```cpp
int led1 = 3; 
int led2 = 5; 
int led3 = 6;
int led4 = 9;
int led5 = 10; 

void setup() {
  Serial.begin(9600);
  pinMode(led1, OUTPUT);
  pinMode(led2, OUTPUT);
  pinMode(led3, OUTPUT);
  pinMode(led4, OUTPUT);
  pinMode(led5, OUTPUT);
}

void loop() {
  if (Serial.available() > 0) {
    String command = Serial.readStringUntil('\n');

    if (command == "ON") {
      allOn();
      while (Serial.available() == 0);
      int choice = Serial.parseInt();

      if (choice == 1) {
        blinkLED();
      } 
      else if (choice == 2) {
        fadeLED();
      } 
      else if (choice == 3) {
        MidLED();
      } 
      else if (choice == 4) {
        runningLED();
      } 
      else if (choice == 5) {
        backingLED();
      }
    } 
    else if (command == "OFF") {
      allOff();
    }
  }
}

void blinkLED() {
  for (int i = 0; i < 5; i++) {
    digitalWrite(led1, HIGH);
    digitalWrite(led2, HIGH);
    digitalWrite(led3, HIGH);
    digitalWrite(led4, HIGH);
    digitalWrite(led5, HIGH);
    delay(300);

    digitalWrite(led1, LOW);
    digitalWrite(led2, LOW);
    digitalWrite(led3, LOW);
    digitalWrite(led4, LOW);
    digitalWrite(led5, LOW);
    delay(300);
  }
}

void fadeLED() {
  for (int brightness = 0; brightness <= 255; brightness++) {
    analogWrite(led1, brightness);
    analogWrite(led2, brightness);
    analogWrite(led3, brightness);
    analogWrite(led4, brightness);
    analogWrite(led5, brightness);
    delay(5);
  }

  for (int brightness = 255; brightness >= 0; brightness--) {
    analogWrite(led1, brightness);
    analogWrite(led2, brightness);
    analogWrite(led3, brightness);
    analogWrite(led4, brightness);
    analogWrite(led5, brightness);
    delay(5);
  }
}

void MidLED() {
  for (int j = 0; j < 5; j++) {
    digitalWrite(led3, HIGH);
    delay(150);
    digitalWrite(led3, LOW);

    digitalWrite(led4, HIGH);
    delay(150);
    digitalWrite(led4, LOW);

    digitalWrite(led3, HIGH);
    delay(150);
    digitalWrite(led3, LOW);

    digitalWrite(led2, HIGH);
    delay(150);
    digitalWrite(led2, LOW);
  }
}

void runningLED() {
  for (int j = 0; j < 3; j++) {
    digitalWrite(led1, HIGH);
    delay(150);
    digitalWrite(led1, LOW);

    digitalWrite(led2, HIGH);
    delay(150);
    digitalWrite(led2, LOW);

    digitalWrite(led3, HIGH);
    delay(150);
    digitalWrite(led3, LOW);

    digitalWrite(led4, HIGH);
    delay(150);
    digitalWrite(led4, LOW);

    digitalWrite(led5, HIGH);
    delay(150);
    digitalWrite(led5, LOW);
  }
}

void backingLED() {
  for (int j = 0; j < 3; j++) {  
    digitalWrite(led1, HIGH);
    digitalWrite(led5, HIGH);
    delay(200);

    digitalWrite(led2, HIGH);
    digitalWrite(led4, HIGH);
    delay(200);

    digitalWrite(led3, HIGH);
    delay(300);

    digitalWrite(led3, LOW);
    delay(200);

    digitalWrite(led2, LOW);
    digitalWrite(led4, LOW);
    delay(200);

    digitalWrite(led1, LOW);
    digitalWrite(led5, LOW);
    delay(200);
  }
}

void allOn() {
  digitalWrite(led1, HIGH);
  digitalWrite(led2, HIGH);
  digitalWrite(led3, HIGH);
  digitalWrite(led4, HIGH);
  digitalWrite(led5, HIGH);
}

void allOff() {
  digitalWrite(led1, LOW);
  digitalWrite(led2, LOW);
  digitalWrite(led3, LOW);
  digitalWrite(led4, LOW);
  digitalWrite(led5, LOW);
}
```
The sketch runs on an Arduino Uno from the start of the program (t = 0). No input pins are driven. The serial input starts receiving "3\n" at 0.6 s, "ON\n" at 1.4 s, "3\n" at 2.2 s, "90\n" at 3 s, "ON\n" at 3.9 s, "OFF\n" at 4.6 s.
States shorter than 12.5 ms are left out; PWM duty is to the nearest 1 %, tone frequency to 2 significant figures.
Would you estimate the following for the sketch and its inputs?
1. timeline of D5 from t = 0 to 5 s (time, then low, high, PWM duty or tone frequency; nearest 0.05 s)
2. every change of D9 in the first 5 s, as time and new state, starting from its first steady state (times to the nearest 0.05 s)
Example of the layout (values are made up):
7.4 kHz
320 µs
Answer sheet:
0 s low; 1.4 s high; 2.8 s low; 3.25 s high; 3.4 s low; 3.85 s high; 4 s low; 4.45 s high; 4.6 s low
0 s low; 1.4 s high; 2.5 s low; 2.95 s high; 3.1 s low; 3.55 s high; 3.7 s low; 4.15 s high; 4.3 s low; 4.75 s high; 4.9 s low
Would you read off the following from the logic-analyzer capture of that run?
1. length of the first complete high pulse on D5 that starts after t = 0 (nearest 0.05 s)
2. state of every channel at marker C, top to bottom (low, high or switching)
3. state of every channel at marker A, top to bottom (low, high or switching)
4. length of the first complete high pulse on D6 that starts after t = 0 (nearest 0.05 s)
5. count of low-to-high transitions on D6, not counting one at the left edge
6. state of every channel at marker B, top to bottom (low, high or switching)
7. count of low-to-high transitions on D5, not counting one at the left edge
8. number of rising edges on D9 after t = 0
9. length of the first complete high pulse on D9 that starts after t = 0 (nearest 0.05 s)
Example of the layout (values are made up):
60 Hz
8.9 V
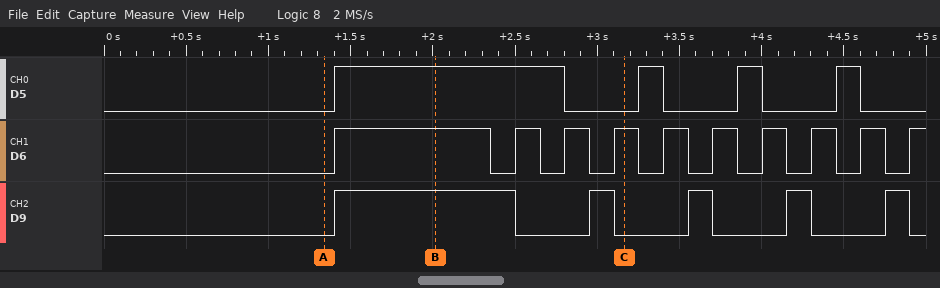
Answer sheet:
1.40 s
D5 low, D6 high, D9 low
D5 low, D6 low, D9 low
0.95 s
10
D5 high, D6 high, D9 high
4
5
1.10 s
